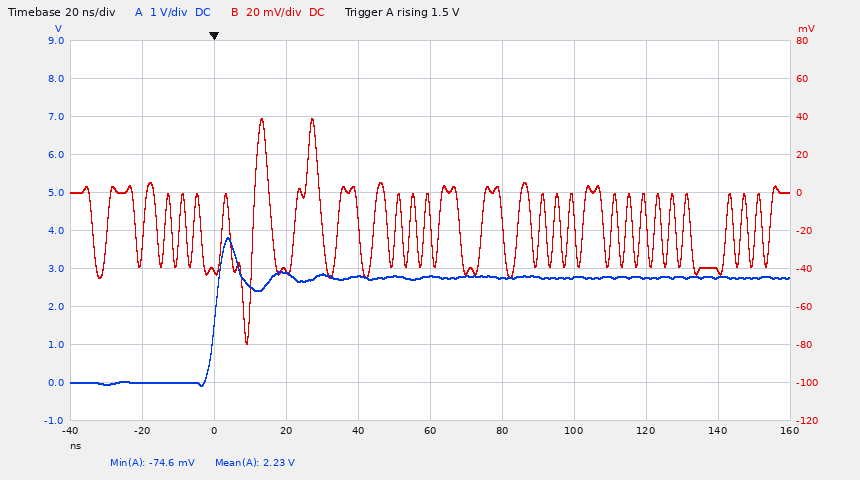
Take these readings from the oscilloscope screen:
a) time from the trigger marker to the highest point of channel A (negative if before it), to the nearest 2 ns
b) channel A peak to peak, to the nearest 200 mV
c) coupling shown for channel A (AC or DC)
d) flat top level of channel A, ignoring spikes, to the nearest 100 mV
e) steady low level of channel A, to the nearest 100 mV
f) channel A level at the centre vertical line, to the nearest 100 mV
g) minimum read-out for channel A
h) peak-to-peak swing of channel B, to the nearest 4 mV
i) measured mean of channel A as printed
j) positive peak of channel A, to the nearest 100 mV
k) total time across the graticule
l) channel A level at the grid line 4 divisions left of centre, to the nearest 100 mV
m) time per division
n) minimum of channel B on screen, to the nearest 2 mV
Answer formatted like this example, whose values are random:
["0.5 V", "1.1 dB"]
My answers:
["+4 ns", "3.8 V", "DC", "2.8 V", "0.0 V", "2.8 V", "-74.6 mV", "120 mV", "2.23 V", "3.8 V", "200 ns", "0.0 V", "20 ns", "-80 mV"]
